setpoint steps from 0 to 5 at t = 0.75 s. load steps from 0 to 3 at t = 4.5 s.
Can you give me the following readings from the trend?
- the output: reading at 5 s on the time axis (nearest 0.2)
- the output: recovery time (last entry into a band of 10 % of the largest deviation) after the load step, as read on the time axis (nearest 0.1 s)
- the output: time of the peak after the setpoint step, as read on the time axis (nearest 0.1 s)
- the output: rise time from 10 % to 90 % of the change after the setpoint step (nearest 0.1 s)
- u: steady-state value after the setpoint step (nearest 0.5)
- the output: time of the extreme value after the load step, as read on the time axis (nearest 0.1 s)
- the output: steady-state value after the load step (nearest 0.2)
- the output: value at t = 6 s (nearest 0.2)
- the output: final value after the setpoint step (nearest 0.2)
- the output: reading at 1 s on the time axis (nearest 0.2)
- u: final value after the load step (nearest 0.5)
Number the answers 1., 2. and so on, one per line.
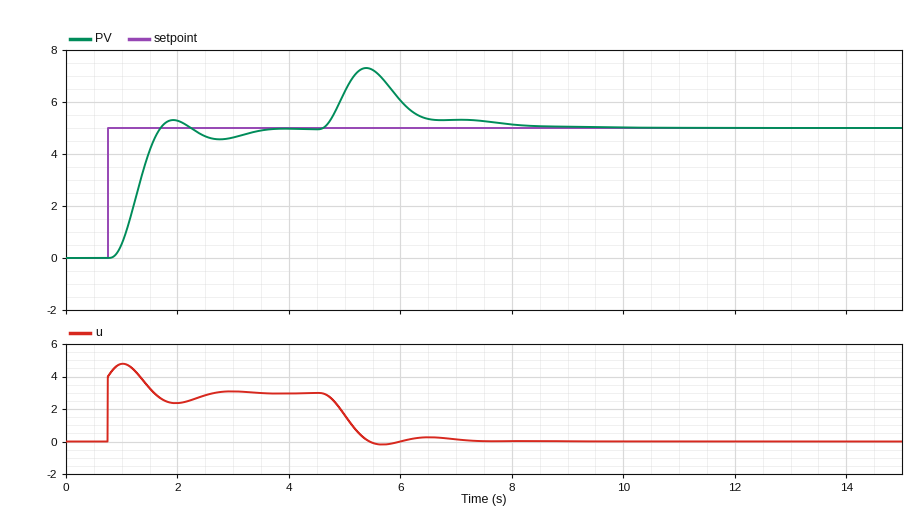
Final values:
1. 6.4
2. 7.6 s
3. 1.9 s
4. 0.6 s
5. 3.0
6. 5.4 s
7. 5.0
8. 6.0
9. 5.0
10. 0.6
11. 0.0
